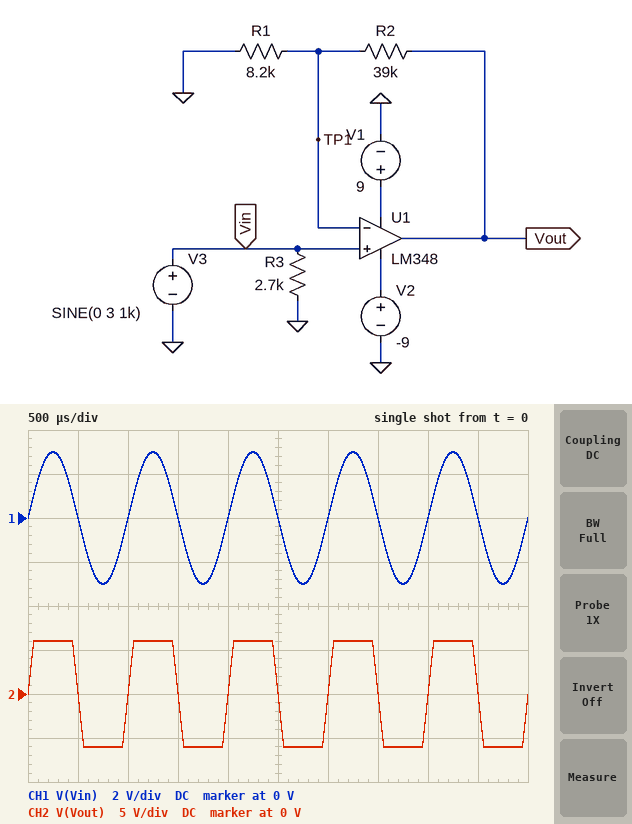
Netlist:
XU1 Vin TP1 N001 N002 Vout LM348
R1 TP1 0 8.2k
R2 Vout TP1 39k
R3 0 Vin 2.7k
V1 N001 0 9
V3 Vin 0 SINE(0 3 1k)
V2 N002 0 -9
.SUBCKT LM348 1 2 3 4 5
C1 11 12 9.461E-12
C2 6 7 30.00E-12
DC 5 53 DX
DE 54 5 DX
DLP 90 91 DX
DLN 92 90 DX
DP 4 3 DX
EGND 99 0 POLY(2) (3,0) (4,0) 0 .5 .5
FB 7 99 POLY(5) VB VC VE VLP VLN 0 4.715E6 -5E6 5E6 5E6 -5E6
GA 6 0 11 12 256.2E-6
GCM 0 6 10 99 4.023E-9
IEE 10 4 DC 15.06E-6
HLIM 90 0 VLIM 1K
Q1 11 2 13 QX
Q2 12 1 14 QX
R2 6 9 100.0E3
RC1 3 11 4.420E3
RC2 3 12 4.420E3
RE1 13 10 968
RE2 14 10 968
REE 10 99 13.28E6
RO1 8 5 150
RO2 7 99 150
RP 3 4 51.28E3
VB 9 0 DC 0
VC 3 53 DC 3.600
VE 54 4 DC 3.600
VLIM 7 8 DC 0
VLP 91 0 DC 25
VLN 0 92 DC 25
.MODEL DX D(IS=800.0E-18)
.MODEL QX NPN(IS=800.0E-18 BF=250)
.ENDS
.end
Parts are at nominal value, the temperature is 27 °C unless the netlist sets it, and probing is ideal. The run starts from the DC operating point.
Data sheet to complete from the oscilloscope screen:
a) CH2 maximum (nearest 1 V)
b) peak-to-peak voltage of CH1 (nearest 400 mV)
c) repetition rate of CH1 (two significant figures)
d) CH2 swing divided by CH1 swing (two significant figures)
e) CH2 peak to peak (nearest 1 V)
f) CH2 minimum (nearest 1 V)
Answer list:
6 V
6.0 V
1.0 kHz
2.0
12 V
-6 V
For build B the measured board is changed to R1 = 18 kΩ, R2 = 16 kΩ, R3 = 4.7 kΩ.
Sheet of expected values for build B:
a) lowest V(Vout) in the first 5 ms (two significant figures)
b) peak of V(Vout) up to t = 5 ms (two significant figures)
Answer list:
-5.7 V
5.7 V
